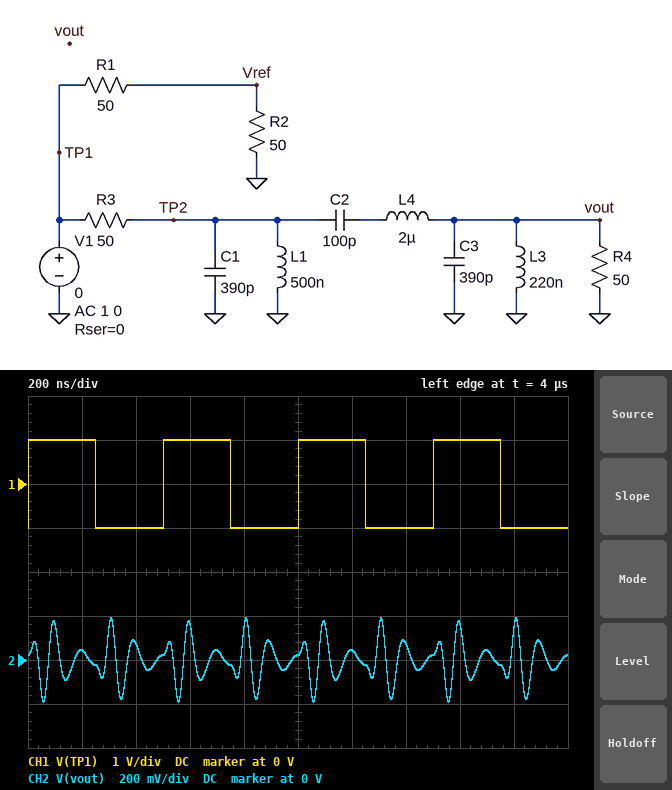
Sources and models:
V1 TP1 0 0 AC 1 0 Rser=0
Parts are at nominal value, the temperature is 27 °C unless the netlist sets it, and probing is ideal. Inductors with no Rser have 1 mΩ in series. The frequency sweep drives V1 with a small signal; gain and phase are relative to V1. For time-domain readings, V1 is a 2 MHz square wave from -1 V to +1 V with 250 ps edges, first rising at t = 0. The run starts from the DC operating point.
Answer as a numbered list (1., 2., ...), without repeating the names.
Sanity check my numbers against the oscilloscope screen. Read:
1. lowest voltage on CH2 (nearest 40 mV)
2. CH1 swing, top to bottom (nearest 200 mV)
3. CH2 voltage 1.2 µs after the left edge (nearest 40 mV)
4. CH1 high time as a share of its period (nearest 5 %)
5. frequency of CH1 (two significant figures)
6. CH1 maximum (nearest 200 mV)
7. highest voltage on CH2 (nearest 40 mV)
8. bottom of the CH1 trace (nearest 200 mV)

1. -200 mV
2. 2.0 V
3. 40 mV
4. 50 %
5. 2.0 MHz
6. 1.0 V
7. 200 mV
8. -1.0 V
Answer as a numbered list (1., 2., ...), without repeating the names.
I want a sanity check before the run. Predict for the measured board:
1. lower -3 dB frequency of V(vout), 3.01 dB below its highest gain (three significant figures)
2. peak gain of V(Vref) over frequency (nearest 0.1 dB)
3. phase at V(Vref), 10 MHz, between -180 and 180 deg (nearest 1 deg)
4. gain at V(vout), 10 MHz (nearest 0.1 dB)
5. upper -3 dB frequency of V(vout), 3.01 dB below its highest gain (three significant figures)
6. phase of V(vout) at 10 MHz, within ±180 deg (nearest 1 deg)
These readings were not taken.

1. 8.85 MHz
2. -6.0 dB
3. 0 deg
4. -9.1 dB
5. 17.2 MHz
6. 87 deg
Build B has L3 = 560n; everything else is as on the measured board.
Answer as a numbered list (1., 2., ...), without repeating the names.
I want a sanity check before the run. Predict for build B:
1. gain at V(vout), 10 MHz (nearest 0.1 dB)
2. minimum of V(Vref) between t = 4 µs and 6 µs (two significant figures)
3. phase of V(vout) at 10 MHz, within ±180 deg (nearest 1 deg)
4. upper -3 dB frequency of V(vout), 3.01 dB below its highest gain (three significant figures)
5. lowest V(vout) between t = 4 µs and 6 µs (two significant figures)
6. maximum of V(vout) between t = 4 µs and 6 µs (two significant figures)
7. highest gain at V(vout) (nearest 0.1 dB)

1. -6.1 dB
2. -500 mV
3. 36 deg
4. 15.9 MHz
5. -250 mV
6. 250 mV
7. -6.0 dB
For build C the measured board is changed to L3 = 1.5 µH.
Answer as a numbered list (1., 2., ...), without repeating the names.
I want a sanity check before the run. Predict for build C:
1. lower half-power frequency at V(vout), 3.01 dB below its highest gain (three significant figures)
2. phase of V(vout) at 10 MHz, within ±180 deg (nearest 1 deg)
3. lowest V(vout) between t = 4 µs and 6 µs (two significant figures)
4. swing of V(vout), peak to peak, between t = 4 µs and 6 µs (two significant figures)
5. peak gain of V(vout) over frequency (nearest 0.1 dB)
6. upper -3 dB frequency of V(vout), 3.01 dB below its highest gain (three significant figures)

1. 8.34 MHz
2. 13 deg
3. -270 mV
4. 530 mV
5. -6.6 dB
6. 15.5 MHz
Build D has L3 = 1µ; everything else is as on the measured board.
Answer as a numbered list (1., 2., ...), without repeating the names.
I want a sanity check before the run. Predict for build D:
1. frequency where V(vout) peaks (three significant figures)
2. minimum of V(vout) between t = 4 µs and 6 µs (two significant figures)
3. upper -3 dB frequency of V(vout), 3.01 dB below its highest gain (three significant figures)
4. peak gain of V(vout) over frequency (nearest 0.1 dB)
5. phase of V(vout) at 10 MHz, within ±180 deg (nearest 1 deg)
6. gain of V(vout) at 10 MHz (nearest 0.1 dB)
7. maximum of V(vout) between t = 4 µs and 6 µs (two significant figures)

1. 12.9 MHz
2. -260 mV
3. 15.6 MHz
4. -6.3 dB
5. 19 deg
6. -6.7 dB
7. 260 mV
